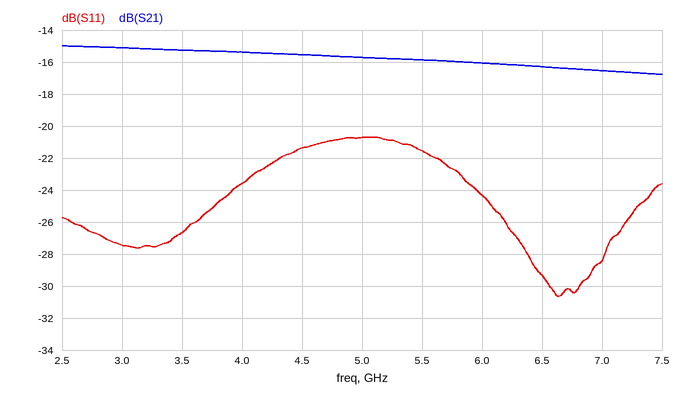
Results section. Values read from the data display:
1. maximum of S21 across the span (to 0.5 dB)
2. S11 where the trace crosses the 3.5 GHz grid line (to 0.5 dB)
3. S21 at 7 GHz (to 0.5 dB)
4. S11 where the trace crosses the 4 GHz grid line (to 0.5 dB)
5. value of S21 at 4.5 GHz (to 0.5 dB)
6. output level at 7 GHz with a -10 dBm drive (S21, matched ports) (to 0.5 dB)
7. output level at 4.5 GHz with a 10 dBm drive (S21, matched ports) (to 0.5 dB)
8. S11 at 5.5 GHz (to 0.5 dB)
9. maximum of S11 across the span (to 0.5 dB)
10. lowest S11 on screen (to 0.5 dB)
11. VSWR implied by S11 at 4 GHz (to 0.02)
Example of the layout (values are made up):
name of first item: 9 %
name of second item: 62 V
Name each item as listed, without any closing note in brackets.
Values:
maximum of S21 across the span: -15.0 dB
S11 where the trace crosses the 3.5 GHz grid line: -26.5 dB
S21 at 7 GHz: -16.5 dB
S11 where the trace crosses the 4 GHz grid line: -23.5 dB
value of S21 at 4.5 GHz: -15.5 dB
output level at 7 GHz with a -10 dBm drive (S21, matched ports): -26.5 dBm
output level at 4.5 GHz with a 10 dBm drive (S21, matched ports): -5.5 dBm
S11 at 5.5 GHz: -21.5 dB
maximum of S11 across the span: -20.5 dB
lowest S11 on screen: -30.5 dB
VSWR implied by S11 at 4 GHz: 1.14
